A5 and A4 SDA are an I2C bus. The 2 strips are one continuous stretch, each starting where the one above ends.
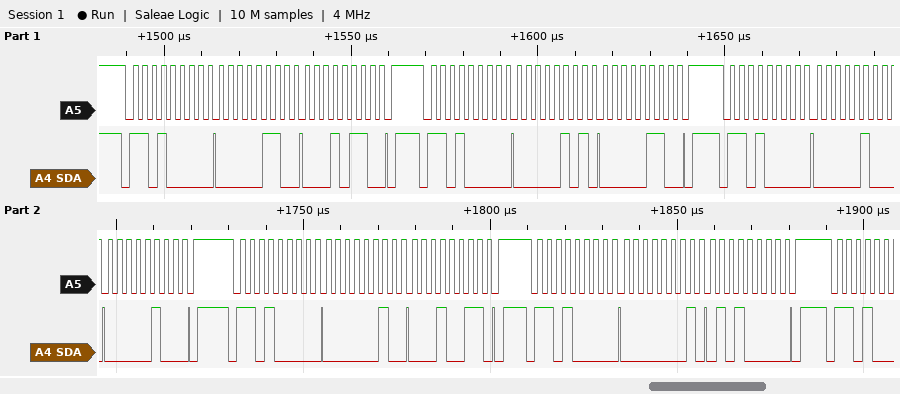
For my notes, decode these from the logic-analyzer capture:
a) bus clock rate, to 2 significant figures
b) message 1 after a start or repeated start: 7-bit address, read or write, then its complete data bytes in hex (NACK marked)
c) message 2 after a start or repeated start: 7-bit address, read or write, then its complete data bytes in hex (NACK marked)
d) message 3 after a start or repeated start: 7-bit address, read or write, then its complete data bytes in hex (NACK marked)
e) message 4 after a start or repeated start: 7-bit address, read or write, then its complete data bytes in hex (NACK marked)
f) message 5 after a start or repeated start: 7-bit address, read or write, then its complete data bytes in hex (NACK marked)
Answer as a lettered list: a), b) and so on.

a) 400 kHz
b) 0x68 write: 06 16
c) 0x68 write: 05 06
d) 0x68 write: 04 04
e) 0x68 write: 02 13
f) 0x68 write: 01 50
